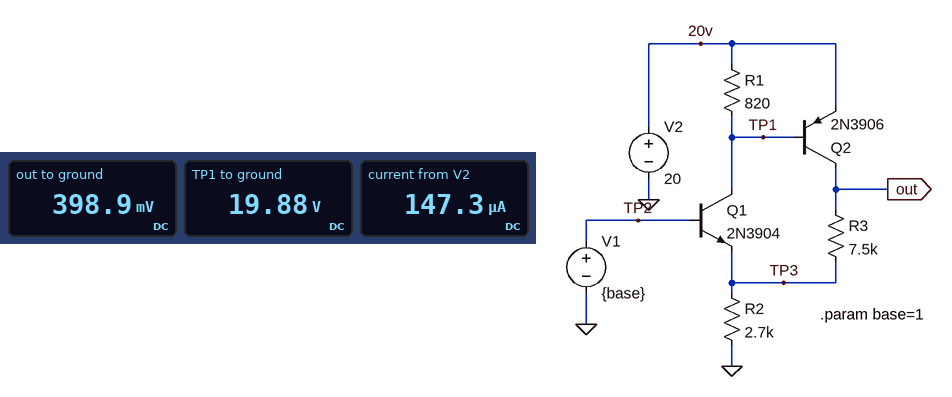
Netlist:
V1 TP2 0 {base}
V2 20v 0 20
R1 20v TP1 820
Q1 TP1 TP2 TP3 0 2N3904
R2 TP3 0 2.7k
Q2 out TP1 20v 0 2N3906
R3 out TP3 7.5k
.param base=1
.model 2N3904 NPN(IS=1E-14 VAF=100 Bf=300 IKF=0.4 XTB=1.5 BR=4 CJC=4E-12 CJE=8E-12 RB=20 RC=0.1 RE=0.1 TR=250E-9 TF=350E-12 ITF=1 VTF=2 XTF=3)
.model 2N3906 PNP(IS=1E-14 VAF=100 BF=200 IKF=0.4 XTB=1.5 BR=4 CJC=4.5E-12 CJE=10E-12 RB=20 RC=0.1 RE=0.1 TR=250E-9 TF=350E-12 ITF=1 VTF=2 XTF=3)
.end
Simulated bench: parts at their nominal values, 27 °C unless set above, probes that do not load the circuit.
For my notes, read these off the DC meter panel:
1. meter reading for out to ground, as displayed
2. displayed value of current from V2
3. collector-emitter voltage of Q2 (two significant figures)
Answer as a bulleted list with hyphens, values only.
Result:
- 398.9 mV
- 147.3 µA
- -20 V
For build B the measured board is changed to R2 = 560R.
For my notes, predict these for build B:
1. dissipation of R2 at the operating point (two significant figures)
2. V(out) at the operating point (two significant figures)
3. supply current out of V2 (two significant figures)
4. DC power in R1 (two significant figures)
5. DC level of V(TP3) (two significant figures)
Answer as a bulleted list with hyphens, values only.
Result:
- 230 µW
- 410 mV
- 640 µA
- 330 µW
- 360 mV
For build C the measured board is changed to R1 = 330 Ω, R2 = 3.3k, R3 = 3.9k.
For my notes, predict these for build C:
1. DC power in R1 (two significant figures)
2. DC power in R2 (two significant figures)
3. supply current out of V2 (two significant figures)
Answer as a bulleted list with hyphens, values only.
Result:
- 4.9 µW
- 49 µW
- 120 µA
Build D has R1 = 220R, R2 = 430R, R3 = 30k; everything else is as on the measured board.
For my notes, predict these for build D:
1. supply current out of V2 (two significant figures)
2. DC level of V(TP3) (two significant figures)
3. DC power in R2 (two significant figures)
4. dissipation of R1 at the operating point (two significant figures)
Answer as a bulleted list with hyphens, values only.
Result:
- 820 µA
- 350 mV
- 290 µW
- 150 µW
